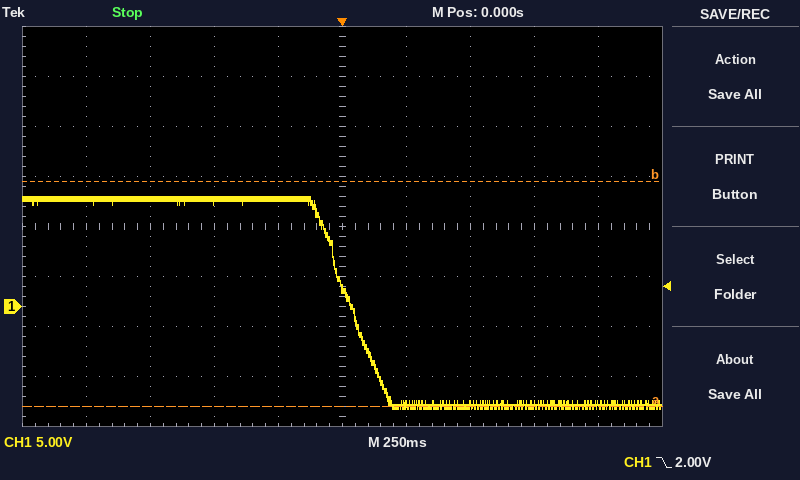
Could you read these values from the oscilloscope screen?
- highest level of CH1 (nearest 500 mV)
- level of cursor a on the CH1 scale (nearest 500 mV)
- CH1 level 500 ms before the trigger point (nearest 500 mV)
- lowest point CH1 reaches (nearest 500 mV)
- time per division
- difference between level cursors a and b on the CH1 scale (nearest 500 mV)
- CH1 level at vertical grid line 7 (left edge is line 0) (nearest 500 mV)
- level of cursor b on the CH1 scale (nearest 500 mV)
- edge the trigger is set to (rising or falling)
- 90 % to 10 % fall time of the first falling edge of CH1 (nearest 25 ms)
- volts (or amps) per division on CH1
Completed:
11.0 V
-10.0 V
10.5 V
-10.0 V
250 ms
22.5 V
-10.0 V
12.5 V
falling
250 ms
5 V
